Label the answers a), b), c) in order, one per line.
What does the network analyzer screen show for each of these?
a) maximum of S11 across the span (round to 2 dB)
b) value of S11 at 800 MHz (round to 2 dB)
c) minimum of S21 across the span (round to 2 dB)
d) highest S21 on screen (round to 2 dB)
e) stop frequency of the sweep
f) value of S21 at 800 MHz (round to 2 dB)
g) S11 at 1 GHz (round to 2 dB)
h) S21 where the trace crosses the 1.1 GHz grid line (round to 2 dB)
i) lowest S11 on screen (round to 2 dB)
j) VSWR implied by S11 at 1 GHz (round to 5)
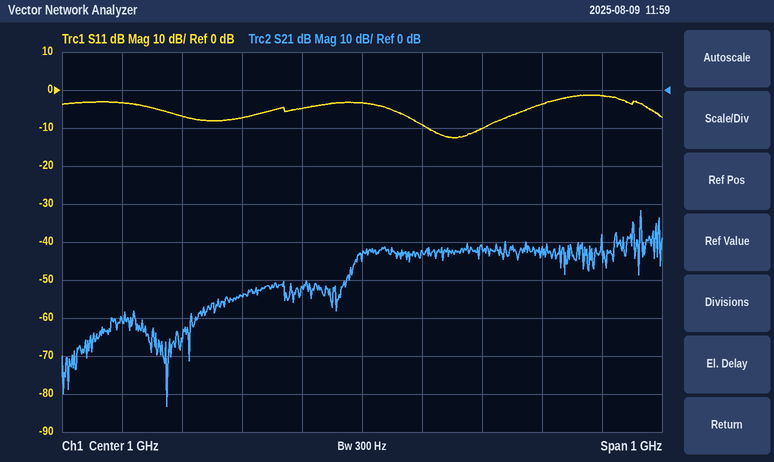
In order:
a) -2 dB
b) -8 dB
c) -84 dB
d) -32 dB
e) 1.5 GHz
f) -54 dB
g) -4 dB
h) -42 dB
i) -12 dB
j) 5
